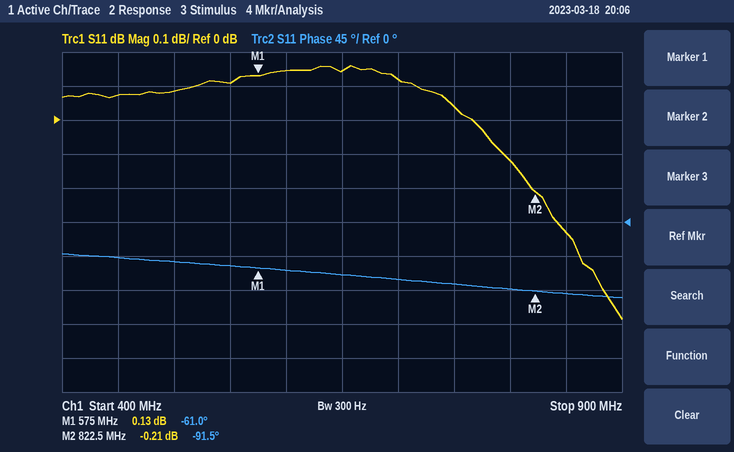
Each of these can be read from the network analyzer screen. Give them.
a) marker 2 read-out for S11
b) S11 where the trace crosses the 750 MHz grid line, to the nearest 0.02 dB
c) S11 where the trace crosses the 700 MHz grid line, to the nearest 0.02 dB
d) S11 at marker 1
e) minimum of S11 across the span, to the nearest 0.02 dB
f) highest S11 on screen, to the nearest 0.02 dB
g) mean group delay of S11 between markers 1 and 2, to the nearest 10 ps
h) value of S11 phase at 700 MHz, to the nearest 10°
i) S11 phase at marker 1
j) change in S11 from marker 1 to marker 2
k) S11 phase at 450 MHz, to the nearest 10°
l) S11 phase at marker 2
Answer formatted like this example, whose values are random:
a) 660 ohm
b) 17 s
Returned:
a) -0.21 dB
b) 0.04 dB
c) 0.12 dB
d) 0.13 dB
e) -0.58 dB
f) 0.16 dB
g) 340 ps
h) -80°
i) -61.0°
j) -0.34 dB
k) -50°
l) -91.5°
